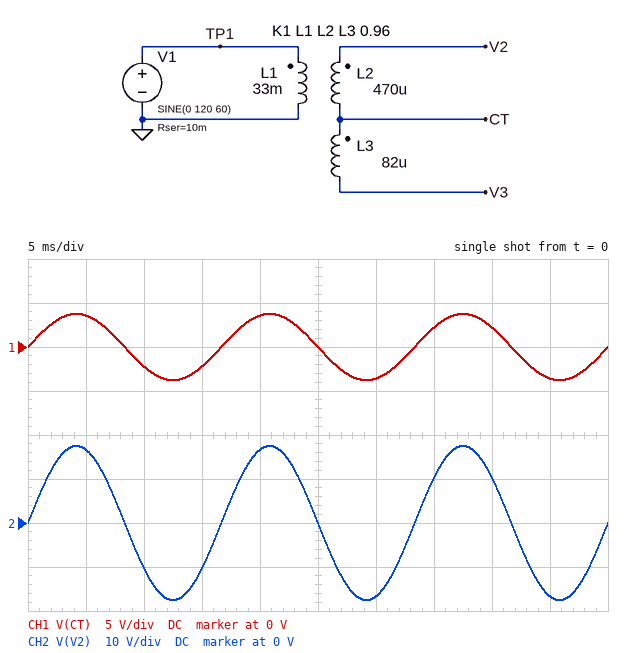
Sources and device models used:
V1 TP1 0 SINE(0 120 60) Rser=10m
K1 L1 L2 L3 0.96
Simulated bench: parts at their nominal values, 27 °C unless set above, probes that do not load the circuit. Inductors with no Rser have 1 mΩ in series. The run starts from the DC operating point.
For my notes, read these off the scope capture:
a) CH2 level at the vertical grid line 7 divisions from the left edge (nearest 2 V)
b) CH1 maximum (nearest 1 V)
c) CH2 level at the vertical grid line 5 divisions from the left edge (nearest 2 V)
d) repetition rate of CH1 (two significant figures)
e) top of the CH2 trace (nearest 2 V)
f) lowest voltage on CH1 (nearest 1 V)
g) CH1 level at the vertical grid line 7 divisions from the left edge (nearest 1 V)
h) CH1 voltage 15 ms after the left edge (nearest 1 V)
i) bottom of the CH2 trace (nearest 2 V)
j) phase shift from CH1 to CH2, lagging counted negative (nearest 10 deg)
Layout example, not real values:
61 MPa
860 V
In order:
10 V
4 V
0 V
60 Hz
18 V
-4 V
2 V
-2 V
-18 V
0 deg
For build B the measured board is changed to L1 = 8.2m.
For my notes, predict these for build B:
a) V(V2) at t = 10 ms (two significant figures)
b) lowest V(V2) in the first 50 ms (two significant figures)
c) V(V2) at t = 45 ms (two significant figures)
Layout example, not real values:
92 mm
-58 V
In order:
-21 V
-35 V
-34 V
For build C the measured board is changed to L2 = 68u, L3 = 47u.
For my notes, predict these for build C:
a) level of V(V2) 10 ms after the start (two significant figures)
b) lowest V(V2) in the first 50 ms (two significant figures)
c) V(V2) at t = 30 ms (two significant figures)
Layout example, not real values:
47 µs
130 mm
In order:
-4.8 V
-8.1 V
-7.7 V
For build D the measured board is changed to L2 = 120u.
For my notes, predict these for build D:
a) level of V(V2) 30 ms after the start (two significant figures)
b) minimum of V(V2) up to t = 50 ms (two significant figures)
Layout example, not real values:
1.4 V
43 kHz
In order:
-10 V
-11 V
